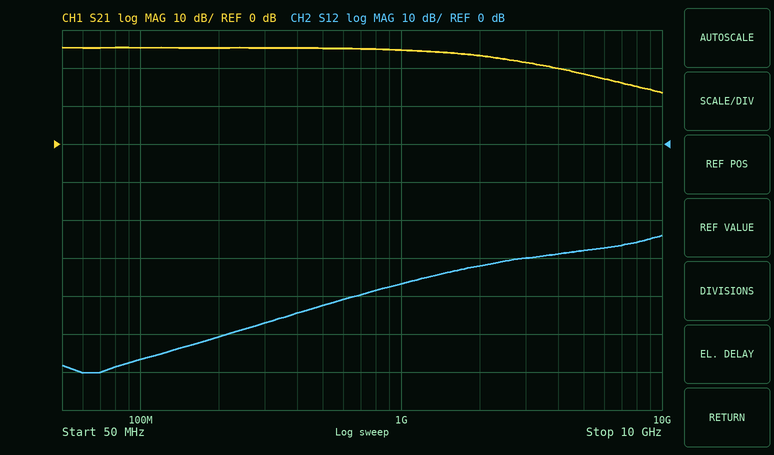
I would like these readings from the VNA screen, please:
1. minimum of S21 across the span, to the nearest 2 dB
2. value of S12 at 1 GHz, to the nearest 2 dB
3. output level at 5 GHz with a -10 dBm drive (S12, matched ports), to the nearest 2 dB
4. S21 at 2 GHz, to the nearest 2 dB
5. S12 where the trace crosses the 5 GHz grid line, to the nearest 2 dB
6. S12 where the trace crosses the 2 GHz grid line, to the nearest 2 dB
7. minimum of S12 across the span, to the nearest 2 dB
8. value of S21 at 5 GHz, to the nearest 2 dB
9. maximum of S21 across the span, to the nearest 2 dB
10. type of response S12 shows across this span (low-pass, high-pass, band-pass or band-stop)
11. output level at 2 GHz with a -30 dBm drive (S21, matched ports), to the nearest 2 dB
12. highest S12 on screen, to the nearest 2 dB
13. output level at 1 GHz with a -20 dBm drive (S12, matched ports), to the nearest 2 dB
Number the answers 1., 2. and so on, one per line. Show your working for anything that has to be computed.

1. 14 dB
2. -36 dB
3. -10 dBm + (-28 dB) = -38 dBm
4. 24 dB
5. -28 dB
6. -32 dB
7. -60 dB
8. 18 dB
9. 26 dB
10. high-pass
11. -30 dBm + (24 dB) = -6 dBm
12. -24 dB
13. -20 dBm + (-36 dB) = -56 dBm
